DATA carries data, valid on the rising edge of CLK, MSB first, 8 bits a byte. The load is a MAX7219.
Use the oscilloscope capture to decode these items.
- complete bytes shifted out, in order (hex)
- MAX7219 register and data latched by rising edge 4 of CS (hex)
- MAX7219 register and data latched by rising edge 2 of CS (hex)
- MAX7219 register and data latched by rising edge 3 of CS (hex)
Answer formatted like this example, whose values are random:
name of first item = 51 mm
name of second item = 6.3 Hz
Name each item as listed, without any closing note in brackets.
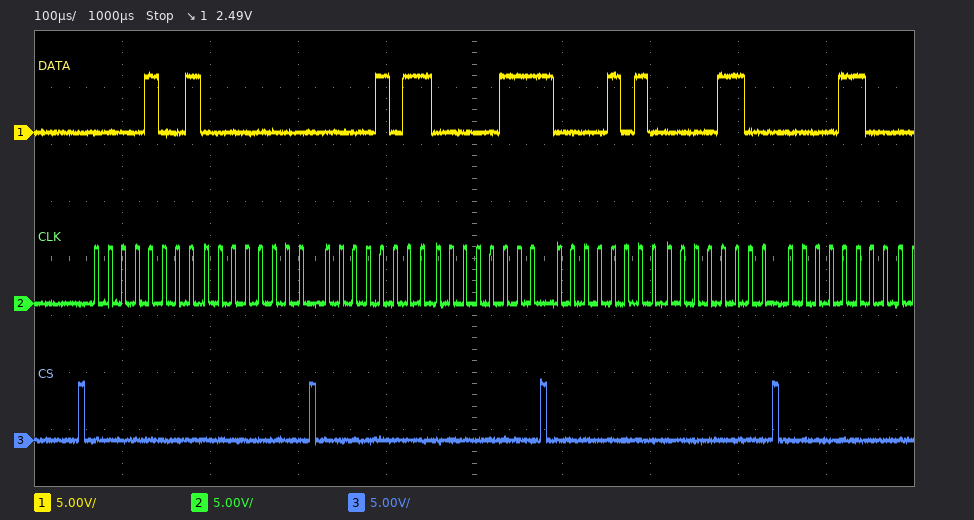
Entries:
complete bytes shifted out, in order = 09 00 0B 07 0A 0C 0C
MAX7219 register and data latched by rising edge 4 of CS = register 0xA, data 0x0C
MAX7219 register and data latched by rising edge 2 of CS = register 0x9, data 0x00
MAX7219 register and data latched by rising edge 3 of CS = register 0xB, data 0x07
